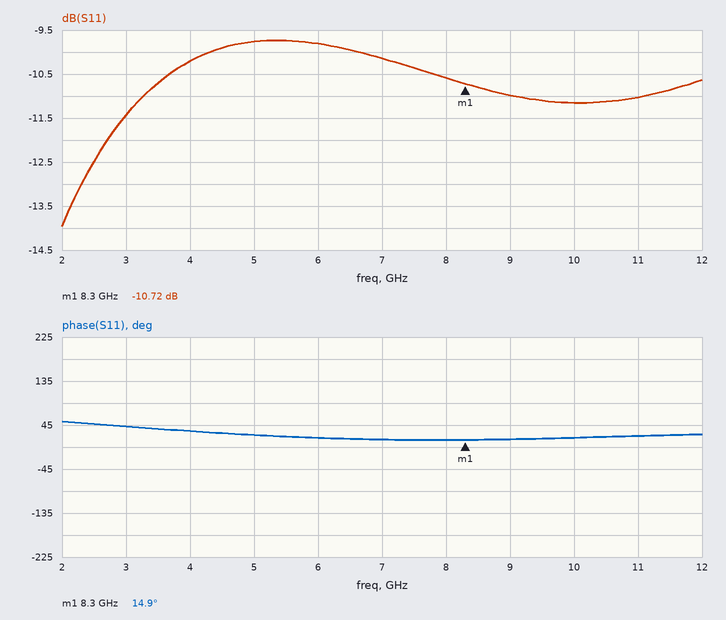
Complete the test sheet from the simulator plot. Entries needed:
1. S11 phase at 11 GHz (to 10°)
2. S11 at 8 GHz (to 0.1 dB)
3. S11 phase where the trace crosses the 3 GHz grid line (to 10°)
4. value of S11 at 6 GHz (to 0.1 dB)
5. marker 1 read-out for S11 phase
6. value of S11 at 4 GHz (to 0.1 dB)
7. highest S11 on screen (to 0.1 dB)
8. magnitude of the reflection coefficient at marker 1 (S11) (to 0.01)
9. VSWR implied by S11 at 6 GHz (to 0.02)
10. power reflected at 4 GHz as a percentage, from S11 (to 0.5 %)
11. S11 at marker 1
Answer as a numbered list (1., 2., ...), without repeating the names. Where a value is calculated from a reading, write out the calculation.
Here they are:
1. 20°
2. -10.6 dB
3. 40°
4. -9.8 dB
5. 14.9°
6. -10.2 dB
7. -9.7 dB
8. 10^(-10.72/20) ≈ 0.29
9. |Γ| = 10^(-9.8/20) = 0.3236; VSWR = (1 + 0.3236)/(1 − 0.3236) ≈ 1.96
10. 10^(-10.2/10) ≈ 9.5 %
11. -10.72 dB
